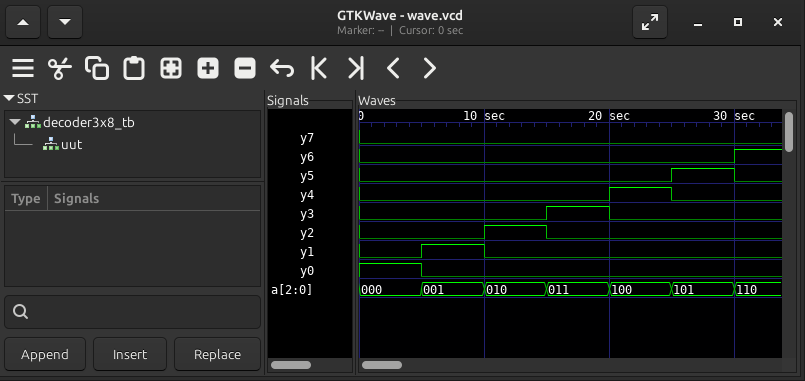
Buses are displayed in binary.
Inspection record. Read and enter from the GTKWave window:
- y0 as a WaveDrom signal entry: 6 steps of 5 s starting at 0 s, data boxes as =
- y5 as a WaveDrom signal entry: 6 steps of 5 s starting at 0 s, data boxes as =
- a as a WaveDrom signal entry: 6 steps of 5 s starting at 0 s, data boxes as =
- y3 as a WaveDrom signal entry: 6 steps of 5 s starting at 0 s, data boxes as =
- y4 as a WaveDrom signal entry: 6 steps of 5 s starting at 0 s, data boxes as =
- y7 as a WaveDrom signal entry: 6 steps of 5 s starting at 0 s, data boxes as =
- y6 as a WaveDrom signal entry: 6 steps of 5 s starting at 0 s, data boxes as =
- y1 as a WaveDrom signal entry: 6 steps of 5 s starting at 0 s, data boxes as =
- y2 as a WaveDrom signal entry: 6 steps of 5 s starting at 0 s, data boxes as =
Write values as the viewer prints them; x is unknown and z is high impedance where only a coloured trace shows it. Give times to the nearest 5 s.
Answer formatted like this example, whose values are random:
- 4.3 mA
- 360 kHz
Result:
- {name: 'y0', wave: '10....'}
- {name: 'y5', wave: '0....1'}
- {name: 'a', wave: '======', data: '000 001 010 011 100 101'}
- {name: 'y3', wave: '0..10.'}
- {name: 'y4', wave: '0...10'}
- {name: 'y7', wave: '0.....'}
- {name: 'y6', wave: '0.....'}
- {name: 'y1', wave: '010...'}
- {name: 'y2', wave: '0.10..'}
